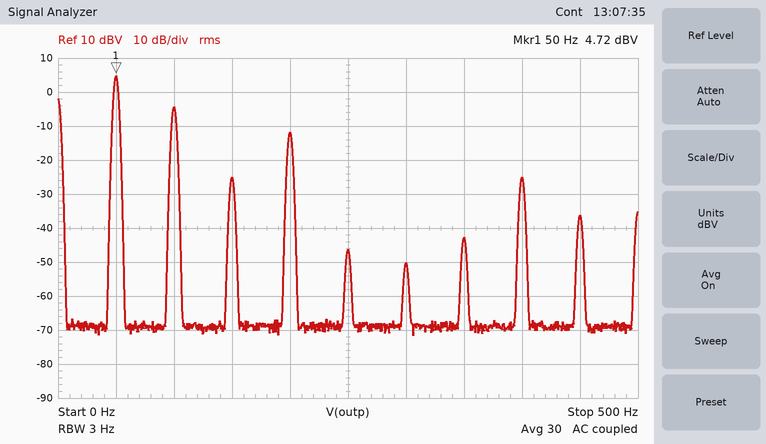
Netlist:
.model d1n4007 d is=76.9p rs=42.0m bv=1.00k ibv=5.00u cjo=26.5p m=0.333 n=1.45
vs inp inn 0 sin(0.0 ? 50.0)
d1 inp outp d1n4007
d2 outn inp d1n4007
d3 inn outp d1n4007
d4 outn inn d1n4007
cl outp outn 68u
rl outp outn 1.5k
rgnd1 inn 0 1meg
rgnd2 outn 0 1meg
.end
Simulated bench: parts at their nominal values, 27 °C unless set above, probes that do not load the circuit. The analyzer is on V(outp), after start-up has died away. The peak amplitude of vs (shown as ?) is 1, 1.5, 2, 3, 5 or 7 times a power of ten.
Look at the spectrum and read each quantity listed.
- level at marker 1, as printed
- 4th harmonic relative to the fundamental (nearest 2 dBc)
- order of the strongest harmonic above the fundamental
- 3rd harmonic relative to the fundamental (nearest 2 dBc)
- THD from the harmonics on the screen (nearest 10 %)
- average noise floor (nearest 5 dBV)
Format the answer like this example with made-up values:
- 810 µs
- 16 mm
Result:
- 4.72 dBV
- -16 dBc
- 2
- -30 dBc
- 40 %
- -70 dBV
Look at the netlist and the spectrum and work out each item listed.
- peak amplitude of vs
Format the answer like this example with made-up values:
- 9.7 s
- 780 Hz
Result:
- 10 V
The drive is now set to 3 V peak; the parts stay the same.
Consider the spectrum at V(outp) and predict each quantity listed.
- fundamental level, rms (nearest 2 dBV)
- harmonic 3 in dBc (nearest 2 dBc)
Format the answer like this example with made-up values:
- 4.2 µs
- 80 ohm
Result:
- -6 dBV
- -22 dBc
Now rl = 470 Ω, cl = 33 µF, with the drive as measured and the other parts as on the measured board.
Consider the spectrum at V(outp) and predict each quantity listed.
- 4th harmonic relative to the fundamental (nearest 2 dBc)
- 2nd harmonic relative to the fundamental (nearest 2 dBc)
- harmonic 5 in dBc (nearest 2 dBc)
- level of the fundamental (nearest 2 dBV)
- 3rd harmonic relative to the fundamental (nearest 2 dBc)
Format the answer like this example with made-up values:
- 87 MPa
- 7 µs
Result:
- -12 dBc
- -12 dBc
- -38 dBc
- 4 dBV
- -32 dBc
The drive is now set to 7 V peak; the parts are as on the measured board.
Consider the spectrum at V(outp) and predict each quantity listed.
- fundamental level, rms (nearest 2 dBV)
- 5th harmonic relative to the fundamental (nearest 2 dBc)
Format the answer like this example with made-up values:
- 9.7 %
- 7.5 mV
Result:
- 2 dBV
- -42 dBc
